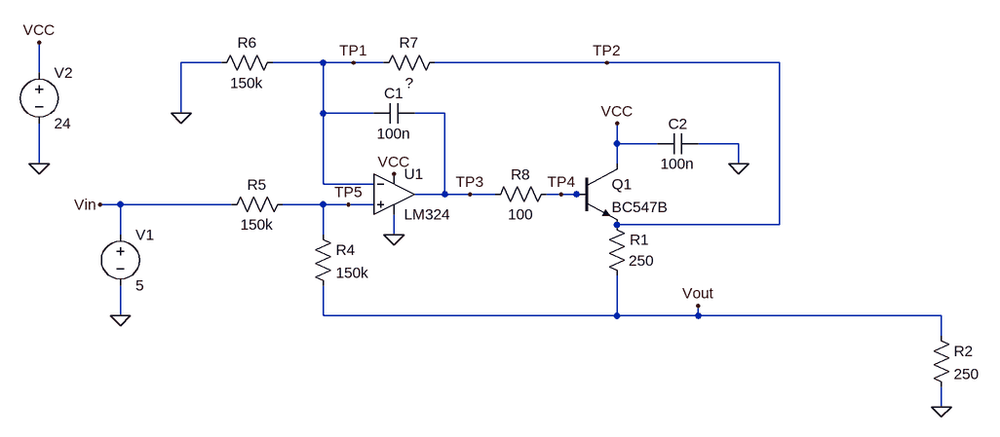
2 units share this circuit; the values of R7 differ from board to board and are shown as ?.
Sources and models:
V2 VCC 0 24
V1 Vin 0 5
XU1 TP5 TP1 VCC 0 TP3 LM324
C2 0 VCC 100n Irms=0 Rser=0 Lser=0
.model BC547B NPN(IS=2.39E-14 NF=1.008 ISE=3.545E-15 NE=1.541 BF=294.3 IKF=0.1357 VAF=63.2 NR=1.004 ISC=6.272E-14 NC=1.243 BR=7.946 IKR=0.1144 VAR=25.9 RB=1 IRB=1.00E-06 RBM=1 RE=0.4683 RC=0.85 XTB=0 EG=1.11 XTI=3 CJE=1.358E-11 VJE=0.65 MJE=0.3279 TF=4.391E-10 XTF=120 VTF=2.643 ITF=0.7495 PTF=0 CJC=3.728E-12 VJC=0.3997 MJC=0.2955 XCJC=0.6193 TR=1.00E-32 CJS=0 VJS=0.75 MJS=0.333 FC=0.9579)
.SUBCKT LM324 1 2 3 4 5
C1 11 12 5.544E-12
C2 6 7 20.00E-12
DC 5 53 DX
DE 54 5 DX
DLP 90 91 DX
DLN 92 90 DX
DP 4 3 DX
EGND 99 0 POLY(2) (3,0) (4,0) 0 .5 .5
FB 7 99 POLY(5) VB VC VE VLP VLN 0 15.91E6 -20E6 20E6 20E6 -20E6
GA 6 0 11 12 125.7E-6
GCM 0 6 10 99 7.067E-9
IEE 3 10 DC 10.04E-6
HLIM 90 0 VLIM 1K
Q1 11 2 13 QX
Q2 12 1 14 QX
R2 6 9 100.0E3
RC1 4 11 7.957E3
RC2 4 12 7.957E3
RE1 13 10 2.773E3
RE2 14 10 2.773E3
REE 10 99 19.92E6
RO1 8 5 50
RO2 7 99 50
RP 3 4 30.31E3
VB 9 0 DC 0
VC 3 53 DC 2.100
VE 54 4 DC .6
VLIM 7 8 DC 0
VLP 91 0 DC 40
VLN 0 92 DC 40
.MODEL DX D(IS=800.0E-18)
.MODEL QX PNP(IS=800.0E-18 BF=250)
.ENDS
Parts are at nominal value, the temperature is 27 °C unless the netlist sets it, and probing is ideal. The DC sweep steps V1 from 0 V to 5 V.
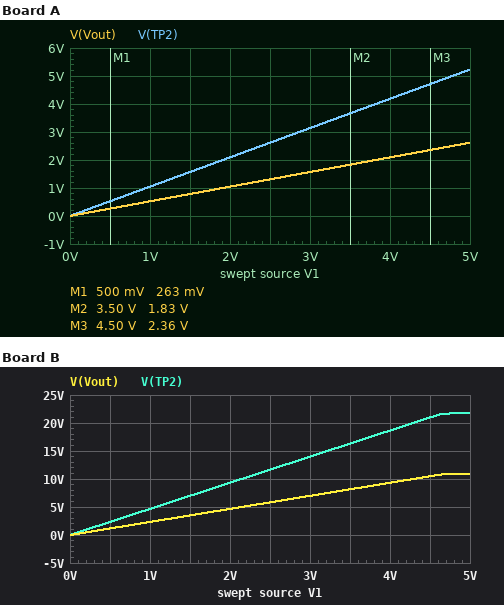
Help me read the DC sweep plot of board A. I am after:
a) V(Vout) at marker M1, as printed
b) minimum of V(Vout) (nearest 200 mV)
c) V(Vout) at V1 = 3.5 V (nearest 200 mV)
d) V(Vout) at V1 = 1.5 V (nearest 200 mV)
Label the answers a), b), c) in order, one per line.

a) 263 mV
b) 0 V
c) 1.8 V
d) 800 mV
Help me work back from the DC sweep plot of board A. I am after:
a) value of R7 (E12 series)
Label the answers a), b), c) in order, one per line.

a) 56 kΩ
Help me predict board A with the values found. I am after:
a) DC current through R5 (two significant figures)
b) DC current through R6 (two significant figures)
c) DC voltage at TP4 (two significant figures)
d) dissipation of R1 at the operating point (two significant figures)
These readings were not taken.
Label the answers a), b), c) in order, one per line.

a) 7.9 µA
b) 25 µA
c) 5.9 V
d) 27 mW
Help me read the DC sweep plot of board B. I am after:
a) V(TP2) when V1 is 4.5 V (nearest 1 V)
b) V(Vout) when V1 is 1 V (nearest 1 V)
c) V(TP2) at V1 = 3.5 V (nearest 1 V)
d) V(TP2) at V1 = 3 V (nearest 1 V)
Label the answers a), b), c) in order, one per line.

a) 21 V
b) 2 V
c) 16 V
d) 14 V
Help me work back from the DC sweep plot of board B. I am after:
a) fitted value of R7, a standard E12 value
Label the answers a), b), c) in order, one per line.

a) 270 kΩ
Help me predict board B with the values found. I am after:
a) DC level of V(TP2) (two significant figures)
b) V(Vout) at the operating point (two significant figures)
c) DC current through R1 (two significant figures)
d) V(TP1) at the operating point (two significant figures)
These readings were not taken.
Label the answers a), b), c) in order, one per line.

a) 22 V
b) 11 V
c) 43 mA
d) 7.8 V
